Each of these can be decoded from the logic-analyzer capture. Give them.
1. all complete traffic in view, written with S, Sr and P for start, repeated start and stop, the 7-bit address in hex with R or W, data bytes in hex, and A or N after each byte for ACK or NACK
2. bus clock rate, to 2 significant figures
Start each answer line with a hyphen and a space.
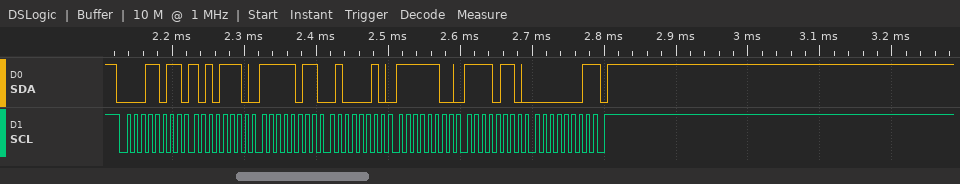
- S 0DR A AE A FB A 42 A FC A F6 A 01 N P
- 100 kHz
